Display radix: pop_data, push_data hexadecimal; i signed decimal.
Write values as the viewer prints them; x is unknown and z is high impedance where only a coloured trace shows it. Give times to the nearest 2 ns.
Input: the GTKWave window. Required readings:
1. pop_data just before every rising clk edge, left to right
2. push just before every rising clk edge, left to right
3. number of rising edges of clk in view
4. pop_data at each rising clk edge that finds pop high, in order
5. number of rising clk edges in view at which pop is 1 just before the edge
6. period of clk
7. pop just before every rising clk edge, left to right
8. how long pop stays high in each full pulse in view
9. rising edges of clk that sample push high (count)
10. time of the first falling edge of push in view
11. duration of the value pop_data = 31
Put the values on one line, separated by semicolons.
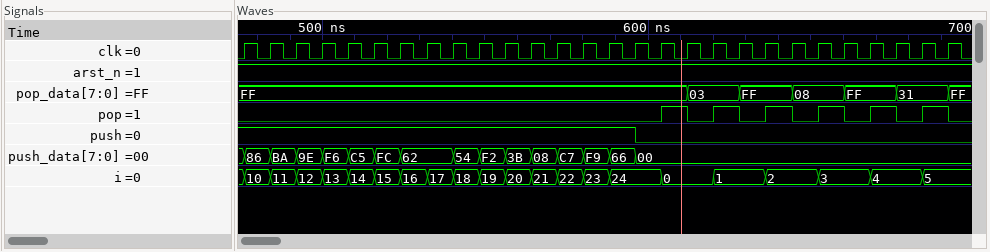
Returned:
FF, FF, FF, FF, FF, FF, FF, FF, FF, FF, FF, FF, FF, FF, FF, FF, FF, FF, 03, 03, FF, FF, 08, 08, FF, FF, 31, 31; 1 1 1 1 1 1 1 1 1 1 1 1 1 1 1 1 0 0 0 0 0 0 0 0 0 0 0 0; 28; FF, 03, FF, 08, FF, 31; 6; 8 ns; 0 0 0 0 0 0 0 0 0 0 0 0 0 0 0 0 0 1 0 1 0 1 0 1 0 1 0 1; 8 ns, 8 ns, 8 ns, 8 ns, 8 ns, 8 ns; 16; 596 ns; 16 ns
